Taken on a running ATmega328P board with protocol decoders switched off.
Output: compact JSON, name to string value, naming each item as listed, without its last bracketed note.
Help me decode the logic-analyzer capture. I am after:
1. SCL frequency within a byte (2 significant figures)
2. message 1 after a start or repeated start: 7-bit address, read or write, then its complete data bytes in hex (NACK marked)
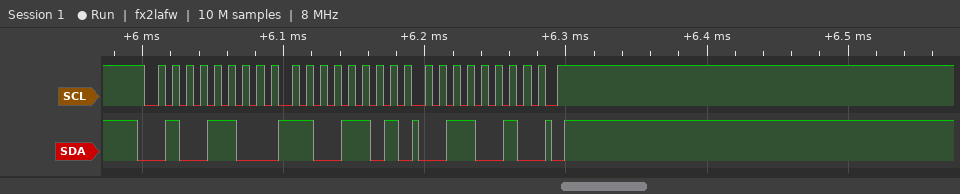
{"SCL frequency within a byte": "100 kHz", "message 1 after a start or repeated start: 7-bit address, read or write, then its complete data bytes in hex": "0x26 write: CD 32"}
